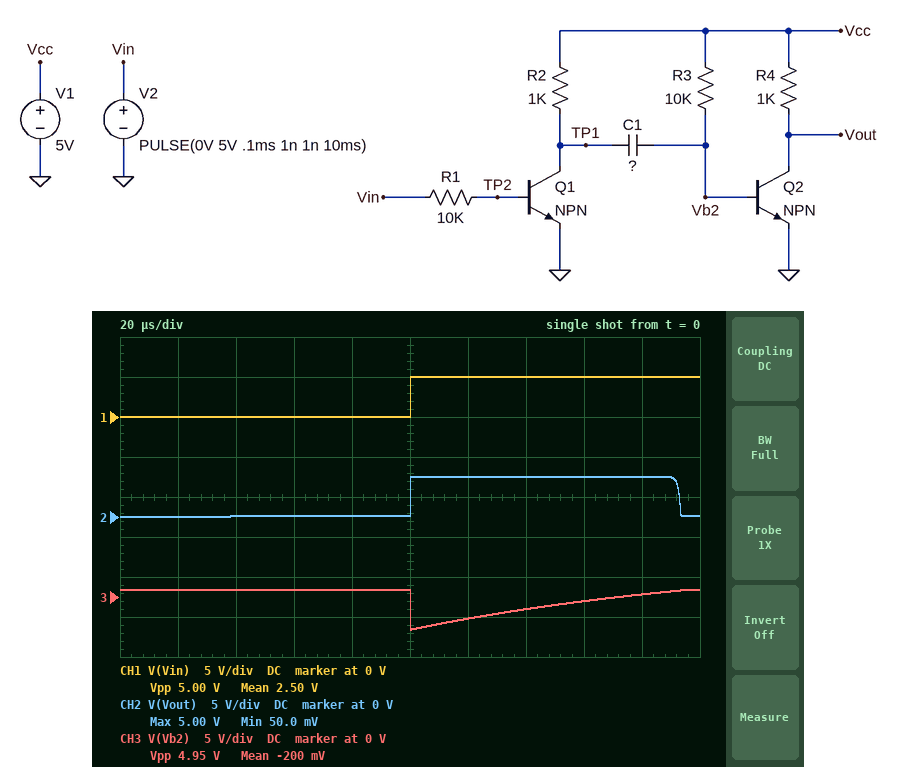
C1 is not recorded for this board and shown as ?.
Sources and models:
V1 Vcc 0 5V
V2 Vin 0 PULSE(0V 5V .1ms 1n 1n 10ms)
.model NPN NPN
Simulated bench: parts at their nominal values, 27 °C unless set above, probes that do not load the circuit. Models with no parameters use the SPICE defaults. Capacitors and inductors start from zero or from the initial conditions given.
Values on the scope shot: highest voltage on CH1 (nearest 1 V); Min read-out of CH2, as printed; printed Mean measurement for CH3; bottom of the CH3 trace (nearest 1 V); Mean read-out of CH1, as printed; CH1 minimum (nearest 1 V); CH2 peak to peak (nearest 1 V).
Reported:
5 V
50.0 mV
-200 mV
-4 V
2.50 V
0 V
5 V
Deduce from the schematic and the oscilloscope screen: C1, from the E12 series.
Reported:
12 nF
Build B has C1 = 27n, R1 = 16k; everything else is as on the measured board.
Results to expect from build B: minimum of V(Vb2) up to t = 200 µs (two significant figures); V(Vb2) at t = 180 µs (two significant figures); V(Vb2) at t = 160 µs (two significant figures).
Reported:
-4.0 V
-1.7 V
-2.2 V
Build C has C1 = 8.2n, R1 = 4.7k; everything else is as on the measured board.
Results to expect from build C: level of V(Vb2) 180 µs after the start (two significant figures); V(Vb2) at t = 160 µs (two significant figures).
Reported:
820 mV
610 mV
